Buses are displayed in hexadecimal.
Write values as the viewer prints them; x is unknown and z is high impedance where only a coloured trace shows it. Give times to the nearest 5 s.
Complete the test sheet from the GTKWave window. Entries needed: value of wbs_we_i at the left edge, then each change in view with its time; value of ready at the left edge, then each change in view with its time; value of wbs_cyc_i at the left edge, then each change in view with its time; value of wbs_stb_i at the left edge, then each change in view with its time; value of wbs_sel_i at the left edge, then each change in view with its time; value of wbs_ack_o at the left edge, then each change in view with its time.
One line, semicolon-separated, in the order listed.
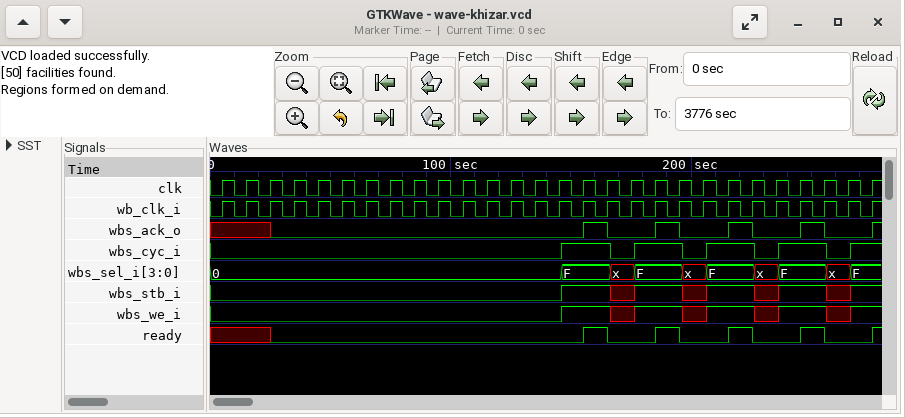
0, 1 at 145 s, x at 165 s, 1 at 175 s, x at 195 s, 1 at 205 s, x at 225 s, 1 at 235 s, x at 255 s, 1 at 265 s; x, 0 at 25 s, 1 at 155 s, 0 at 165 s, 1 at 185 s, 0 at 195 s, 1 at 215 s, 0 at 225 s, 1 at 245 s, 0 at 255 s, 1 at 275 s; 0, 1 at 145 s, 0 at 165 s, 1 at 175 s, 0 at 195 s, 1 at 205 s, 0 at 225 s, 1 at 235 s, 0 at 255 s, 1 at 265 s; 0, 1 at 145 s, x at 165 s, 1 at 175 s, x at 195 s, 1 at 205 s, x at 225 s, 1 at 235 s, x at 255 s, 1 at 265 s; 0, F at 145 s, x at 165 s, F at 175 s, x at 195 s, F at 205 s, x at 225 s, F at 235 s, x at 255 s, F at 265 s; x, 0 at 25 s, 1 at 155 s, 0 at 165 s, 1 at 185 s, 0 at 195 s, 1 at 215 s, 0 at 225 s, 1 at 245 s, 0 at 255 s, 1 at 275 s
